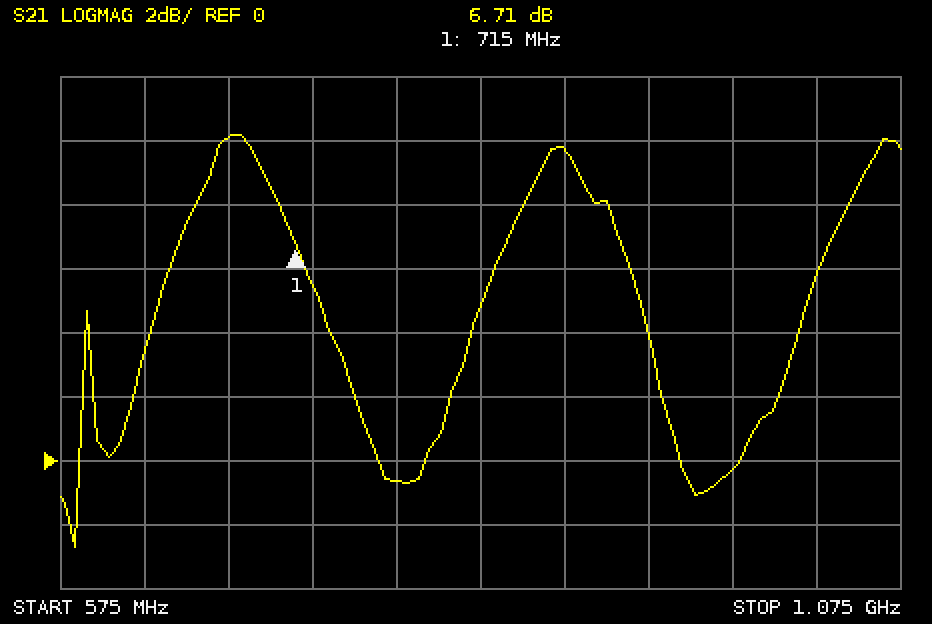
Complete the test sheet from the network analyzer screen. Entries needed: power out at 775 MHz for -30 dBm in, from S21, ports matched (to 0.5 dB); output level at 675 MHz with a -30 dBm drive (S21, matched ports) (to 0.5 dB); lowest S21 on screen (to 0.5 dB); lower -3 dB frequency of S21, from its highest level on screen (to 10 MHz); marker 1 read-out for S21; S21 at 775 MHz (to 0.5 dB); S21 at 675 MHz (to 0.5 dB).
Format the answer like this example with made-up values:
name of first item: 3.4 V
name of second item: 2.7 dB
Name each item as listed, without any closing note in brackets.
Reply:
power out at 775 MHz for -30 dBm in, from S21, ports matched: -30.5 dBm
output level at 675 MHz with a -30 dBm drive (S21, matched ports): -20.0 dBm
lowest S21 on screen: -2.5 dB
lower -3 dB frequency of S21, from its highest level on screen: 650 MHz
marker 1 read-out for S21: 6.71 dB
S21 at 775 MHz: -0.5 dB
S21 at 675 MHz: 10.0 dB
